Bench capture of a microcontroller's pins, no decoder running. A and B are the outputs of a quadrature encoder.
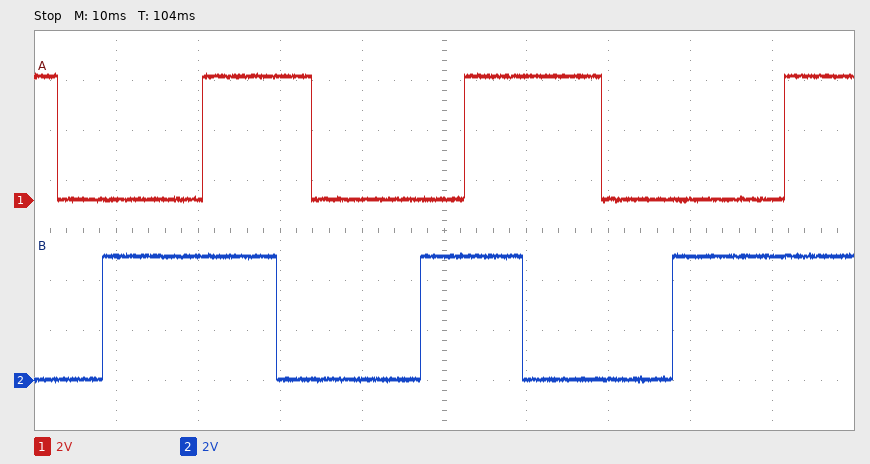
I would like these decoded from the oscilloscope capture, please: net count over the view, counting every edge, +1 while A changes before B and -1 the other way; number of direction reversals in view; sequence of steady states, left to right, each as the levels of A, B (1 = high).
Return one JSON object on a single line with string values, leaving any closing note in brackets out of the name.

{"net count over the view, counting every edge, +1 while A changes before B and -1 the other way": "-11", "number of direction reversals in view": "0", "sequence of steady states, left to right, each as the levels of A, B": "10 00 01 11 10 00 01 11 10 00 01 11"}
